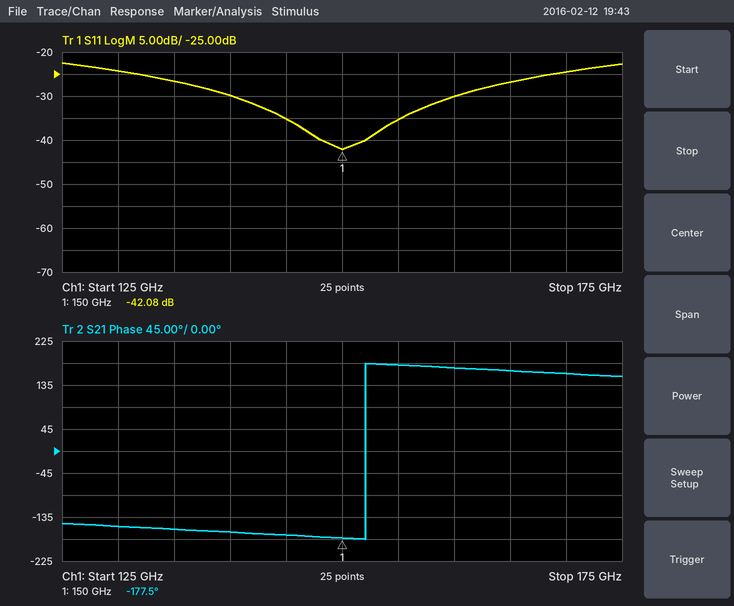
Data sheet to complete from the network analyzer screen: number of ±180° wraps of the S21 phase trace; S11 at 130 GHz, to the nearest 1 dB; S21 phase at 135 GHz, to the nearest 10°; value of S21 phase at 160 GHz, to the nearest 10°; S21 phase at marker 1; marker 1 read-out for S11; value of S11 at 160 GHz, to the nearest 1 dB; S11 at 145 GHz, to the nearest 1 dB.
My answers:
1
-24 dB
-160°
170°
-177.5°
-42.08 dB
-30 dB
-35 dB
